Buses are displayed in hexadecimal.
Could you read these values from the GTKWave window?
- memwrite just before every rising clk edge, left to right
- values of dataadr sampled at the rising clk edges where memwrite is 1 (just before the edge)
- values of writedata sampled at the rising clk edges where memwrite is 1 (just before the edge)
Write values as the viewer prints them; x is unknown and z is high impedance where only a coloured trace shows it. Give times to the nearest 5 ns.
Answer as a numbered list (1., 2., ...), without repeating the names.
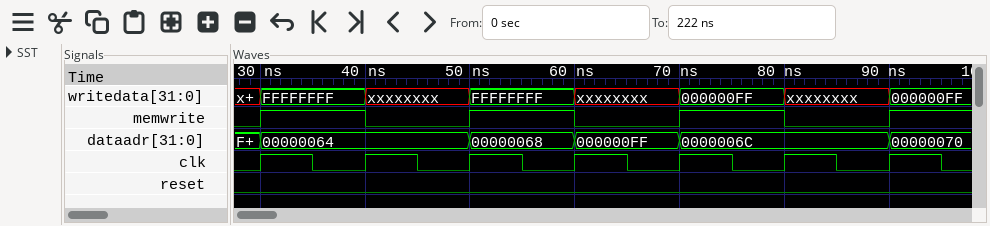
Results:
1. 0 1 0 1 0 1 0
2. 00000064, 00000068, 0000006C
3. FFFFFFFF, FFFFFFFF, 000000FF
